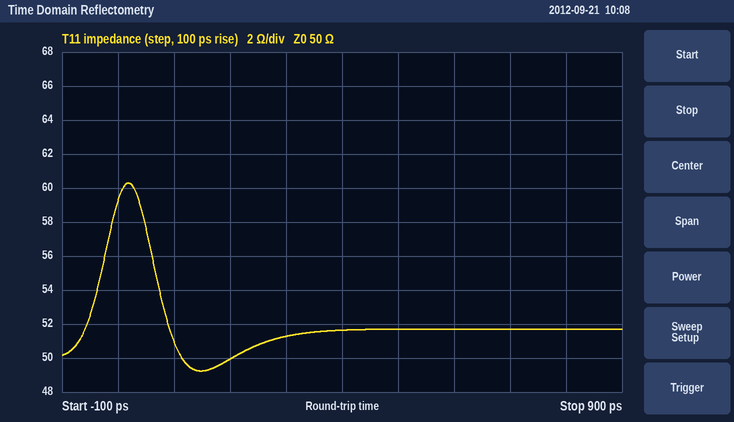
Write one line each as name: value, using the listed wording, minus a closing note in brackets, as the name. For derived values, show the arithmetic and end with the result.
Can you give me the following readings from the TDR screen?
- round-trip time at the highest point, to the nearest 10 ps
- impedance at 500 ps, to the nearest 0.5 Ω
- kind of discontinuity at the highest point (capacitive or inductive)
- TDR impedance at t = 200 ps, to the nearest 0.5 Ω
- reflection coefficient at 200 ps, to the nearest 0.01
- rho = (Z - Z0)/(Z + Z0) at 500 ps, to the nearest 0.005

round-trip time at the highest point, to the nearest 10 ps: 20 ps
impedance at 500 ps, to the nearest 0.5 Ω: 51.5 Ω
kind of discontinuity at the highest point: inductive
TDR impedance at t = 200 ps, to the nearest 0.5 Ω: 50.0 Ω
reflection coefficient at 200 ps, to the nearest 0.01: (50 − 50)/(50 + 50) ≈ 0.00
rho = (Z - Z0)/(Z + Z0) at 500 ps, to the nearest 0.005: (51.5 − 50)/(51.5 + 50) ≈ +0.015
